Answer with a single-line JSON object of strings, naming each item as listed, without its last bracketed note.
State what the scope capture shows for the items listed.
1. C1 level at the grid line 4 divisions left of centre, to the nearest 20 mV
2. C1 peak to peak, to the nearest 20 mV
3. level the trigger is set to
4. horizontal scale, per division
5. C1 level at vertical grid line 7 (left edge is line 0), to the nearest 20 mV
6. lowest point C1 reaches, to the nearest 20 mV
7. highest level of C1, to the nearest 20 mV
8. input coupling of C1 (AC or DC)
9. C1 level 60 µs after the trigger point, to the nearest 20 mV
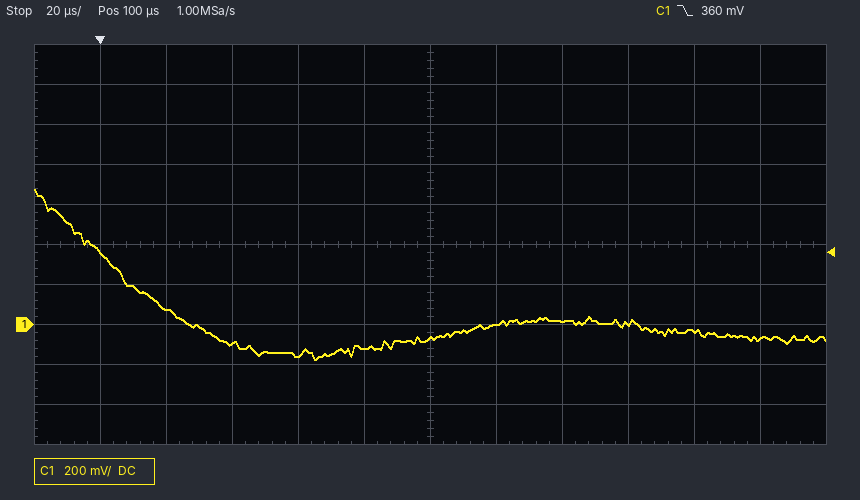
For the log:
{"C1 level at the grid line 4 divisions left of centre, to the nearest 20 mV": "80 mV", "C1 peak to peak, to the nearest 20 mV": "860 mV", "level the trigger is set to": "360 mV", "horizontal scale, per division": "20 µs", "C1 level at vertical grid line 7 (left edge is line 0), to the nearest 20 mV": "0 mV", "lowest point C1 reaches, to the nearest 20 mV": "-180 mV", "highest level of C1, to the nearest 20 mV": "680 mV", "input coupling of C1": "DC", "C1 level 60 µs after the trigger point, to the nearest 20 mV": "-160 mV"}
